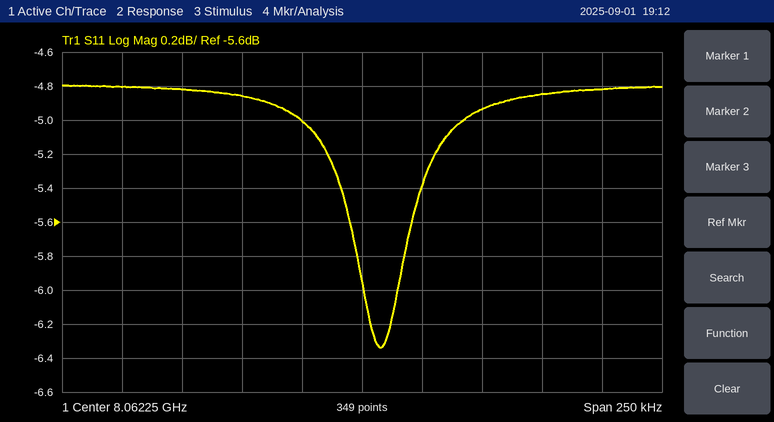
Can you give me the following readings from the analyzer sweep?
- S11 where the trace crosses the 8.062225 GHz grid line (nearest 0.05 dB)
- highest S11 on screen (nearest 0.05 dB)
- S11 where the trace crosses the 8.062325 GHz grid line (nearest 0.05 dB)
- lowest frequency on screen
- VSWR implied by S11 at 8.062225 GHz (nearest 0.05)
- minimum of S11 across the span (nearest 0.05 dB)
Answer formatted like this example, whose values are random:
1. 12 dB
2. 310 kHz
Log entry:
1. -5.00 dB
2. -4.80 dB
3. -4.85 dB
4. 8.062125 GHz
5. 3.55
6. -6.35 dB
